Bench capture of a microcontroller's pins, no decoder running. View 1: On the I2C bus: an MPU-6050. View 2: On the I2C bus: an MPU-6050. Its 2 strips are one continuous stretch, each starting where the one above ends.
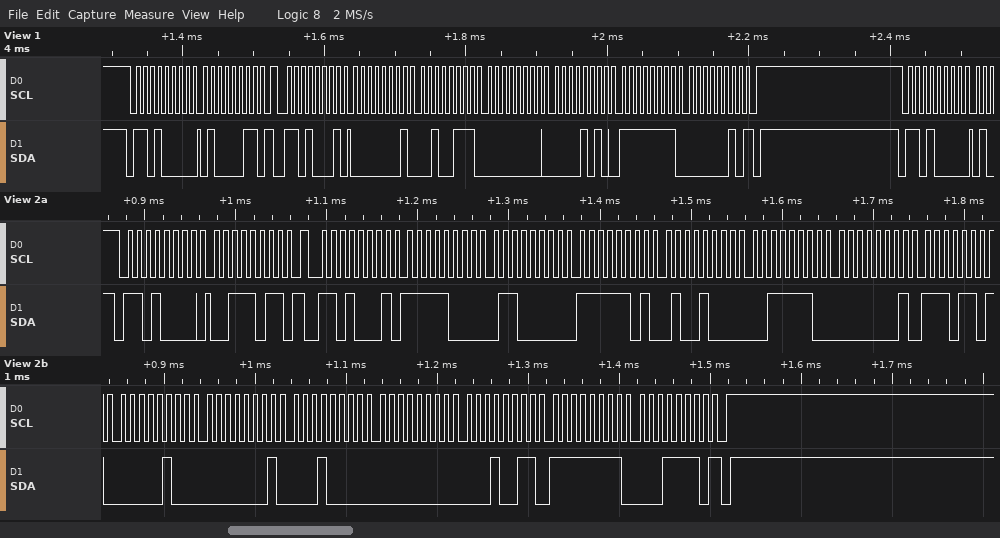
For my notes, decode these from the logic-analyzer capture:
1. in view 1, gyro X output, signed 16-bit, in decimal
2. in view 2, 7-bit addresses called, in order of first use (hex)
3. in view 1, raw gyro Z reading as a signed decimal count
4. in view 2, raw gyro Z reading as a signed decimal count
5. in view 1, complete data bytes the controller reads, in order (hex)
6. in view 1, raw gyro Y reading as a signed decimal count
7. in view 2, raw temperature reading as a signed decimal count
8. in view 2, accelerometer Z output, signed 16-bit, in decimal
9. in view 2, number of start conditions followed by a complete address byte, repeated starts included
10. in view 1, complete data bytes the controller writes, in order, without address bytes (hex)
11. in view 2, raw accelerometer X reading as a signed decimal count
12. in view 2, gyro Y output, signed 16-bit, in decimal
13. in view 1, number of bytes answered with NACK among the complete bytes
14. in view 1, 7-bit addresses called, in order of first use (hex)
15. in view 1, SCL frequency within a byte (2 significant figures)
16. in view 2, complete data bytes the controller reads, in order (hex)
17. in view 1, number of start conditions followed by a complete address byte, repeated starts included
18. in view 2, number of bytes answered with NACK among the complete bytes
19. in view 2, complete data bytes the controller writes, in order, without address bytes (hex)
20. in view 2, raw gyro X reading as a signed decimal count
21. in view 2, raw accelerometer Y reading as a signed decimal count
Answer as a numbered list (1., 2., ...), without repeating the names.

1. 295
2. 0x68
3. -254
4. -226
5. 01 27 00 0A FF 02
6. 10
7. -4860
8. 15873
9. 2
10. 43
11. -1952
12. 19
13. 1
14. 0x68
15. 100 kHz
16. F8 60 FD 48 3E 01 ED 04 01 10 00 13 FF 1E
17. 3
18. 1
19. 3B
20. 272
21. -696
